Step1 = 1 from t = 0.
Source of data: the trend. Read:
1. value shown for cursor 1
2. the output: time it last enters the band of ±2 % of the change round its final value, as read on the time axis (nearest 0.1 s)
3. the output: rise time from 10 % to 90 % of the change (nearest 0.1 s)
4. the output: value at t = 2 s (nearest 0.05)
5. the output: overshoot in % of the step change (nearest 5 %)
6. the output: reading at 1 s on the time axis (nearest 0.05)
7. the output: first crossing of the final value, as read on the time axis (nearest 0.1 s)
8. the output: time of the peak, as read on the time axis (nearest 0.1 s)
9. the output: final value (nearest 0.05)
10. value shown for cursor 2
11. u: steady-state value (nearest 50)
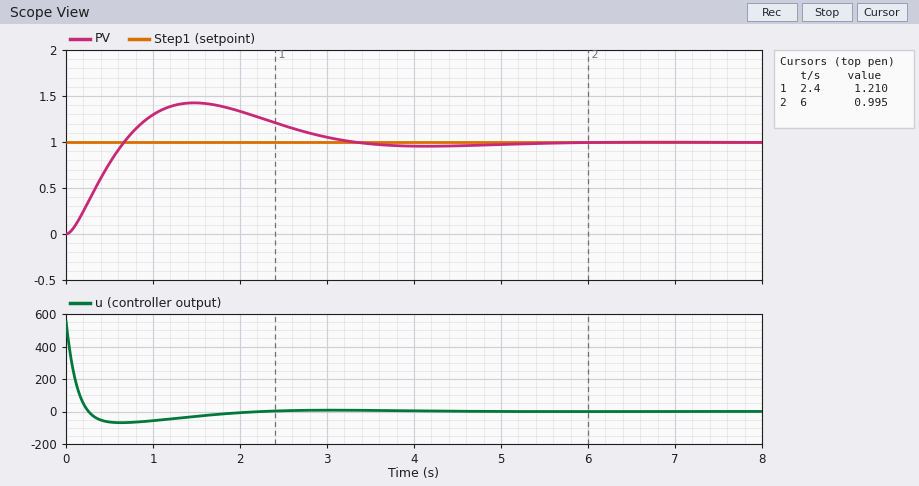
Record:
1.210
5.1 s
0.5 s
1.35
45 %
1.30
0.7 s
1.5 s
1.00
0.995
0
